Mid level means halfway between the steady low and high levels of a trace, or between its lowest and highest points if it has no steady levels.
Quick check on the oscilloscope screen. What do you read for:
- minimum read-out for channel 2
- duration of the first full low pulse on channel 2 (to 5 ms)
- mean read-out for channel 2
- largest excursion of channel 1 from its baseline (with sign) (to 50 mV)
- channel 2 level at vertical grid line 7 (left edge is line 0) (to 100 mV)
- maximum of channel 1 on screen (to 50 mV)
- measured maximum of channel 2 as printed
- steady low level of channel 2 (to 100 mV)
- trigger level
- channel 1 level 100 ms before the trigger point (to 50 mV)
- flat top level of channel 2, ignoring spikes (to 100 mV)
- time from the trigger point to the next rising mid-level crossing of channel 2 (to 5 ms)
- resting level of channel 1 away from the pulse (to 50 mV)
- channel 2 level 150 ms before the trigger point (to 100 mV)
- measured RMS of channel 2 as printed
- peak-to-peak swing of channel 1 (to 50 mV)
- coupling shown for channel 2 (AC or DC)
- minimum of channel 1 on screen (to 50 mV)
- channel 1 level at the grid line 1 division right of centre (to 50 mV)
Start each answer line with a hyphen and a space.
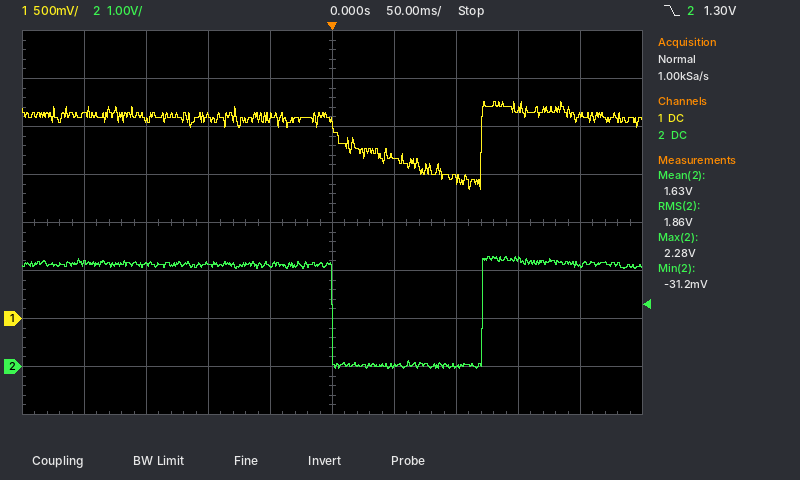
- -31.2 mV
- 120 ms
- 1.63 V
- -750 mV
- 0.0 V
- 2.25 V
- 2.28 V
- 0.0 V
- 1.30 V
- 2.10 V
- 2.1 V
- 120 ms
- 2.10 V
- 2.1 V
- 1.86 V
- 900 mV
- DC
- 1.35 V
- 1.70 V
